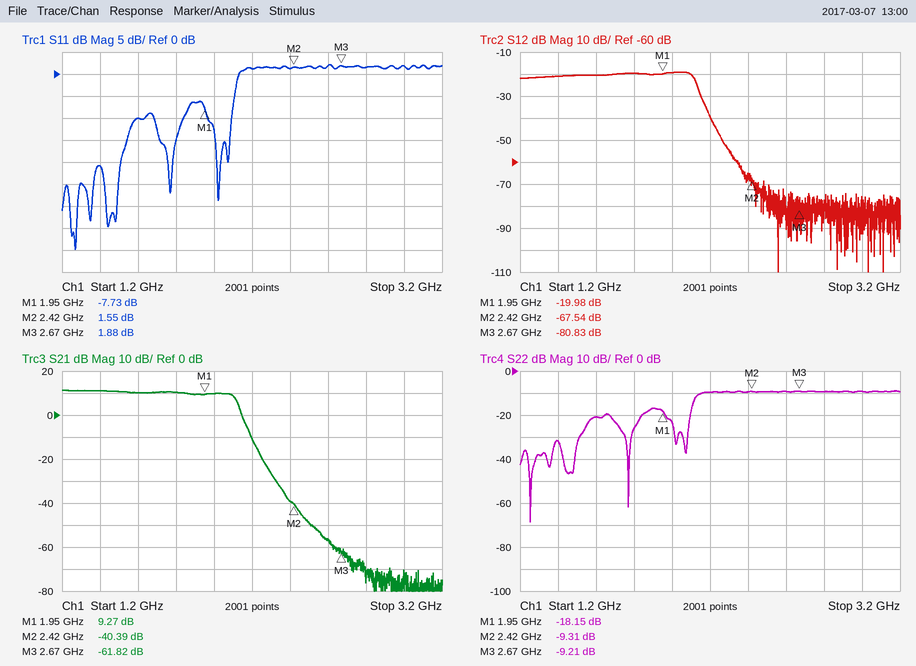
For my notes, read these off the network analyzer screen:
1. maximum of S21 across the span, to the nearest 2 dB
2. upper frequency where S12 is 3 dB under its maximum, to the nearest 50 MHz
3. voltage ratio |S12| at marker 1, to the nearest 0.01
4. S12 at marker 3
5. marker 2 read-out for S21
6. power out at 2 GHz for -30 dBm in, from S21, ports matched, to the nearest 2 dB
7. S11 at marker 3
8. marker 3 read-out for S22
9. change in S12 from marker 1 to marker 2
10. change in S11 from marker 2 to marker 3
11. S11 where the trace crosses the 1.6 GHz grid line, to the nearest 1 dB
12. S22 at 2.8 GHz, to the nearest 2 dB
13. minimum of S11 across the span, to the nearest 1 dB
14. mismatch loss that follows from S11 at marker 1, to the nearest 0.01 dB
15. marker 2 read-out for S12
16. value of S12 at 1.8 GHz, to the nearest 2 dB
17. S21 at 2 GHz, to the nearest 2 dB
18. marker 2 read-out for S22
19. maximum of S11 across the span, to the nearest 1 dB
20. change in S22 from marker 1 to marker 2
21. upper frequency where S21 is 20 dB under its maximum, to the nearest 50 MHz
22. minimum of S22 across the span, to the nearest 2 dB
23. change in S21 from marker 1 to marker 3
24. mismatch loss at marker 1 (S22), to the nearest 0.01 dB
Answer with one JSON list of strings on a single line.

["12 dB", "2.10 GHz", "0.10", "-80.83 dB", "-40.39 dB", "-20 dBm", "1.88 dB", "-9.21 dB", "-47.56 dB", "0.33 dB", "-10 dB", "-10 dB", "-40 dB", "0.80 dB", "-67.54 dB", "-20 dB", "10 dB", "-9.31 dB", "2 dB", "8.84 dB", "2.20 GHz", "-68 dB", "-71.09 dB", "0.07 dB"]
